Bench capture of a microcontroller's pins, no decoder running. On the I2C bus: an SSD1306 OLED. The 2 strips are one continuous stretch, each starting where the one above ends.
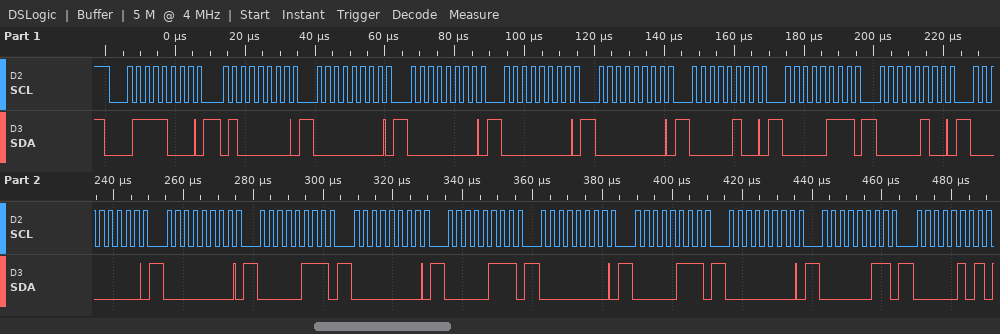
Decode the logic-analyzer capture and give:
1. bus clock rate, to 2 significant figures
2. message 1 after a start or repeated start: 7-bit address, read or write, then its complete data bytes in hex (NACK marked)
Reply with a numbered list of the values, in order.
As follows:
1. 400 kHz
2. 0x3C write: 40 00 00 00 00 04 07 04 00 00 07 00 07 00 07 00 03 05
